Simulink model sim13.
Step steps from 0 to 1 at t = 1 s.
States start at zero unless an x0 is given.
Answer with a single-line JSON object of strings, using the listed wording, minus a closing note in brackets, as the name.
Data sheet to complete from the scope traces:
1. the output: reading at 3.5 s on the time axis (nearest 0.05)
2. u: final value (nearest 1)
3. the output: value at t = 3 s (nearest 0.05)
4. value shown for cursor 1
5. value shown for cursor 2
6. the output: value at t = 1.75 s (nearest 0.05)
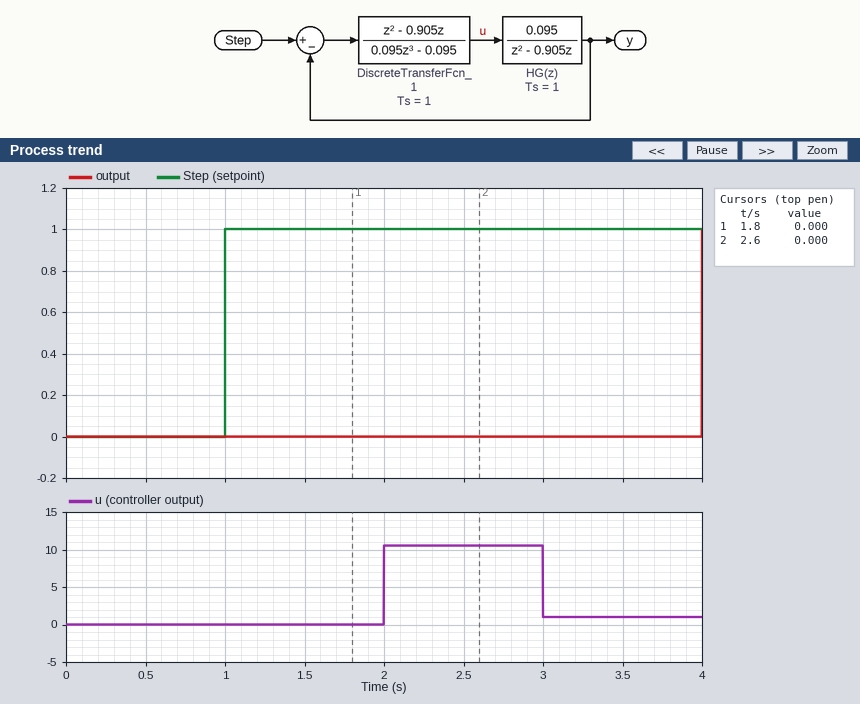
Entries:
{"the output: reading at 3.5 s on the time axis": "0.00", "u: final value": "1", "the output: value at t = 3 s": "0.00", "value shown for cursor 1": "0.000", "value shown for cursor 2": "0.000", "the output: value at t = 1.75 s": "0.00"}
